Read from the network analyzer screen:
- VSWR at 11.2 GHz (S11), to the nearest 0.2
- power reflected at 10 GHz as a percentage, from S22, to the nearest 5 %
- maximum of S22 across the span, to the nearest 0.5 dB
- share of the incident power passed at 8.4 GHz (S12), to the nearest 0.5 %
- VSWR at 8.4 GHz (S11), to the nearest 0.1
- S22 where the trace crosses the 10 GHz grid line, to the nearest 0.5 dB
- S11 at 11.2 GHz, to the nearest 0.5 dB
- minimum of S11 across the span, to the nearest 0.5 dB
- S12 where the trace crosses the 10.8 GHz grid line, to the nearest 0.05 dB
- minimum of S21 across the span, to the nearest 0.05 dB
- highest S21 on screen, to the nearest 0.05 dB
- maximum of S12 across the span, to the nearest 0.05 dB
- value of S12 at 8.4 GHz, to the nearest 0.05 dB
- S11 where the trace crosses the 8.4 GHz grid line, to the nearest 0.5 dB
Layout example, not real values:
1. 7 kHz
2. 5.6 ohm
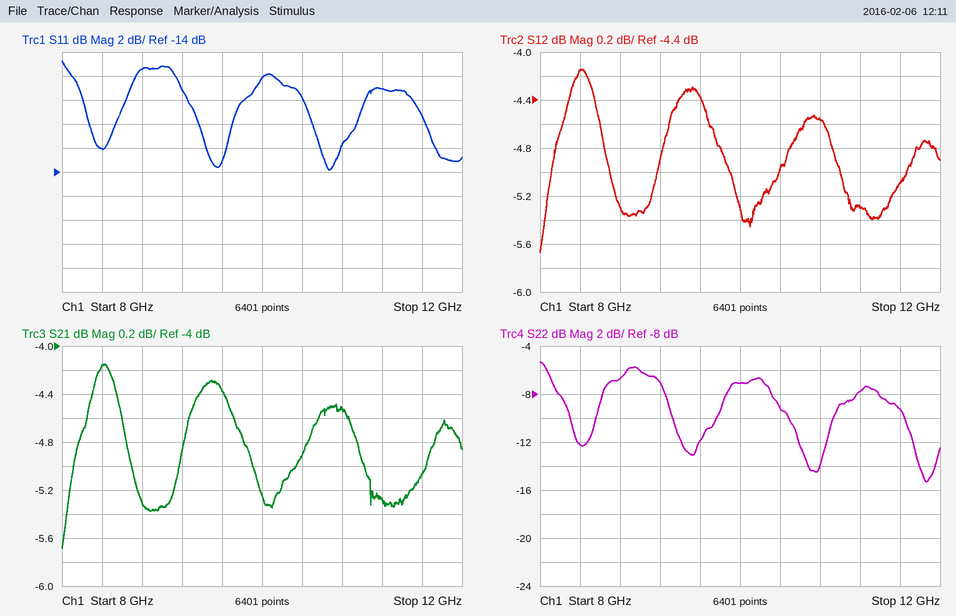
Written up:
1. 2.6
2. 20 %
3. -5.5 dB
4. 38.5 %
5. 1.7
6. -7.0 dB
7. -7.0 dB
8. -14.0 dB
9. -4.55 dB
10. -5.70 dB
11. -4.15 dB
12. -4.15 dB
13. -4.15 dB
14. -12.0 dB
